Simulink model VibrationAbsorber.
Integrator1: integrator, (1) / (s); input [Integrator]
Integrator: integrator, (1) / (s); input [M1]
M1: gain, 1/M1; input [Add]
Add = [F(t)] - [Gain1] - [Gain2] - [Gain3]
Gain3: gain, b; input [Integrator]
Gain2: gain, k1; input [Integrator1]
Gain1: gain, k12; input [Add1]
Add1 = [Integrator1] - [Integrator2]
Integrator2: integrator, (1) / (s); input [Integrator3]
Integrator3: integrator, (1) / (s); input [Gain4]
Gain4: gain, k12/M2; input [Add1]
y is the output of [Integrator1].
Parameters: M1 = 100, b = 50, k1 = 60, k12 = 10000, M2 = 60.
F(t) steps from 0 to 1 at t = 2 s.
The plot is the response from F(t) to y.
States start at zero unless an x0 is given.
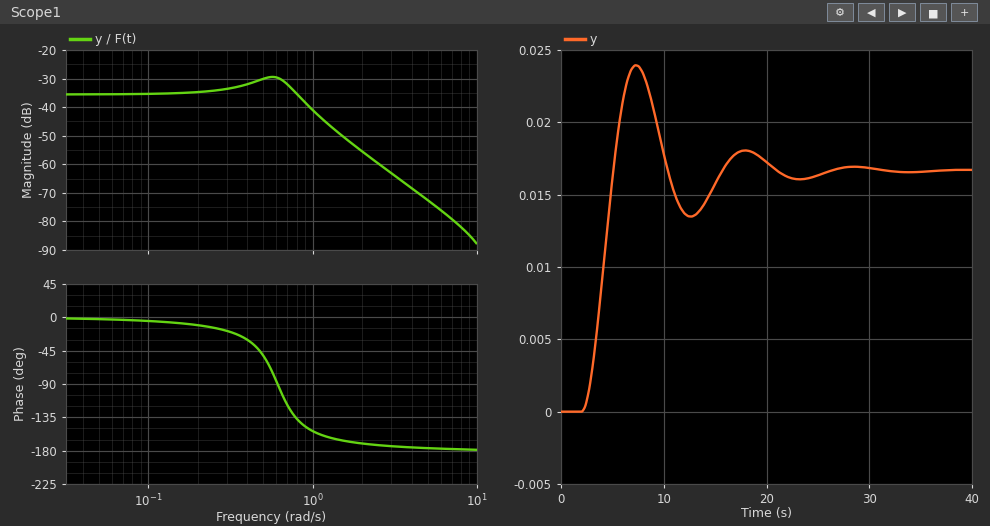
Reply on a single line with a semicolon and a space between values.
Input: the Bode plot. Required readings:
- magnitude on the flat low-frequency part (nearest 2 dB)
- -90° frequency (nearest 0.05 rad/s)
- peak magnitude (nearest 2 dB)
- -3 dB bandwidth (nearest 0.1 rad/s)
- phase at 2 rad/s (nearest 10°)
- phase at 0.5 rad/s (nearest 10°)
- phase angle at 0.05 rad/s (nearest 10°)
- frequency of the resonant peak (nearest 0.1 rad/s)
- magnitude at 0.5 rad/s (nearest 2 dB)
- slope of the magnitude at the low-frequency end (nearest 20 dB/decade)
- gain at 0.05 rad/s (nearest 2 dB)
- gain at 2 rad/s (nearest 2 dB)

-36 dB; 0.60 rad/s; -30 dB; 0.9 rad/s; -170°; -50°; 0°; 0.6 rad/s; -30 dB; 0 dB/decade; -36 dB; -56 dB
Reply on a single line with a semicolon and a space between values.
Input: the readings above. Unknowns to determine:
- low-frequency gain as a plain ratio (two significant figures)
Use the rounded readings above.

0.016
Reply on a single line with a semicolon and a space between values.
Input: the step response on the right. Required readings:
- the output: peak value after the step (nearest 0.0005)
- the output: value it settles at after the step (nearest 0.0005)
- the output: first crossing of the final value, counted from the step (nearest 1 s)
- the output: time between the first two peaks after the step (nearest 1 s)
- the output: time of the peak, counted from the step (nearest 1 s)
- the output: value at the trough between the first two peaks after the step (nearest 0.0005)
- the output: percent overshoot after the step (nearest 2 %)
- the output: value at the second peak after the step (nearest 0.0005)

0.0240; 0.0165; 3 s; 11 s; 5 s; 0.0135; 44 %; 0.0180
